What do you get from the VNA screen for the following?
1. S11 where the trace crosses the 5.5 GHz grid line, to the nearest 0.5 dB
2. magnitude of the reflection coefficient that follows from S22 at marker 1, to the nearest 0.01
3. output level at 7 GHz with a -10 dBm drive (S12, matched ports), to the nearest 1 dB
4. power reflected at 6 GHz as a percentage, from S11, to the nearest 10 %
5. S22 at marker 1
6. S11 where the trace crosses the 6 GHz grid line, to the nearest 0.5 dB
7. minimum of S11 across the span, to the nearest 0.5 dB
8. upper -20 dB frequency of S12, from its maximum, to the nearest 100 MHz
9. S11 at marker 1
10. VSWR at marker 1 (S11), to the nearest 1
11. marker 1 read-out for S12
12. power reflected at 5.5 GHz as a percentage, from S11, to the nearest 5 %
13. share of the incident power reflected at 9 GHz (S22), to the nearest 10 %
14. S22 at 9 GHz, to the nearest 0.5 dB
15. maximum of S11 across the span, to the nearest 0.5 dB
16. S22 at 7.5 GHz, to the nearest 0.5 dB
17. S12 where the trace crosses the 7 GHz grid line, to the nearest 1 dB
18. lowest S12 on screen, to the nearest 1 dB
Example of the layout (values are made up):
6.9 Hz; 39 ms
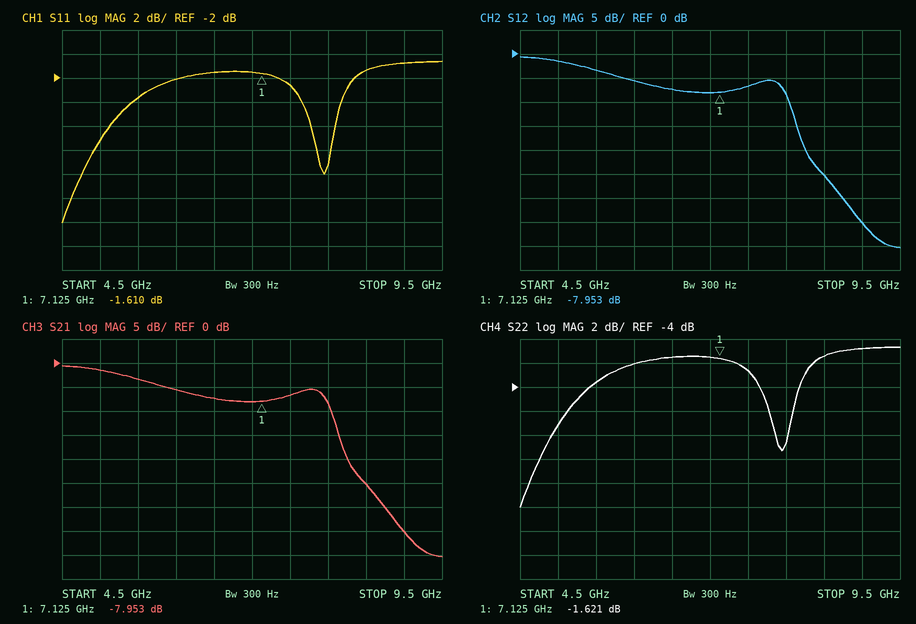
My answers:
-3.5 dB; 0.83; -18 dBm; 60 %; -1.621 dB; -2.0 dB; -14.0 dB; 8.3 GHz; -1.610 dB; 11; -7.953 dB; 45 %; 80 %; -1.0 dB; -0.5 dB; -2.5 dB; -8 dB; -40 dB
